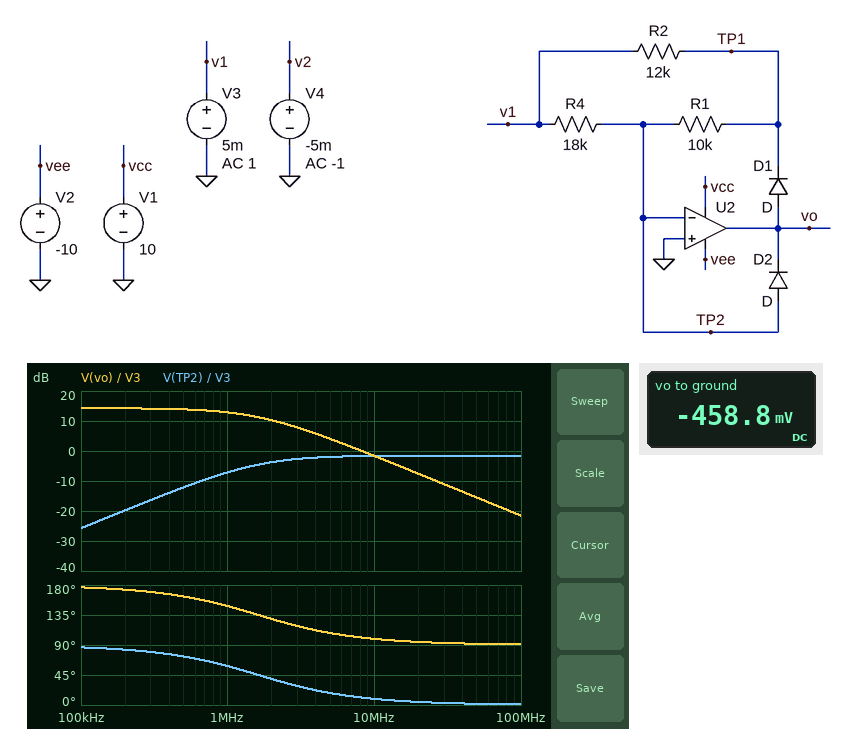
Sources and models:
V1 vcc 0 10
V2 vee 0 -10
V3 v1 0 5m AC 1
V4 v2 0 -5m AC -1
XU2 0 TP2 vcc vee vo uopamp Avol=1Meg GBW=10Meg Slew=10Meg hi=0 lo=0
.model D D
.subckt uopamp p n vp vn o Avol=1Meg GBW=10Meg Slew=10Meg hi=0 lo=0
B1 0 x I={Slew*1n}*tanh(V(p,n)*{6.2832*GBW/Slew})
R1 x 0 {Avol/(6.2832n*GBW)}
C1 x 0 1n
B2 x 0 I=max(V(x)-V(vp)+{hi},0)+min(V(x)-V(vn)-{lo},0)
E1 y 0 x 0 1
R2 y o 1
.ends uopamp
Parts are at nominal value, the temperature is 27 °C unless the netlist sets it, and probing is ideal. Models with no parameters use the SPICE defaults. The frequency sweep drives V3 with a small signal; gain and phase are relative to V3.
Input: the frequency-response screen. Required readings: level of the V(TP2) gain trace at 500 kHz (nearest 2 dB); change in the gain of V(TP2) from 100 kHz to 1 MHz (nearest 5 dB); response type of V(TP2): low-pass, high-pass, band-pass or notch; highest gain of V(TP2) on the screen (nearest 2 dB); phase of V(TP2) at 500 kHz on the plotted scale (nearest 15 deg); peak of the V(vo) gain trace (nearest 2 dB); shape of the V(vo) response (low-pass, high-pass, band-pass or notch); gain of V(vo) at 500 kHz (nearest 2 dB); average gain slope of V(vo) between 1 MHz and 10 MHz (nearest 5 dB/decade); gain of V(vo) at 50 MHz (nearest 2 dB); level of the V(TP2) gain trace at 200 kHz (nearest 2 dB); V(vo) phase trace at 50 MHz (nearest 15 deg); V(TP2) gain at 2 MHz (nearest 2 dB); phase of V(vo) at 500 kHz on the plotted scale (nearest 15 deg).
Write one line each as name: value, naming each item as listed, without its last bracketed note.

level of the V(TP2) gain trace at 500 kHz: -12 dB
change in the gain of V(TP2) from 100 kHz to 1 MHz: 20 dB
response type of V(TP2): low-pass, high-pass, band-pass or notch: high-pass
highest gain of V(TP2) on the screen: -2 dB
phase of V(TP2) at 500 kHz on the plotted scale: 75 deg
peak of the V(vo) gain trace: 14 dB
shape of the V(vo) response: low-pass
gain of V(vo) at 500 kHz: 14 dB
average gain slope of V(vo) between 1 MHz and 10 MHz: -15 dB/decade
gain of V(vo) at 50 MHz: -16 dB
level of the V(TP2) gain trace at 200 kHz: -20 dB
V(vo) phase trace at 50 MHz: 90 deg
V(TP2) gain at 2 MHz: -4 dB
phase of V(vo) at 500 kHz on the plotted scale: 165 deg
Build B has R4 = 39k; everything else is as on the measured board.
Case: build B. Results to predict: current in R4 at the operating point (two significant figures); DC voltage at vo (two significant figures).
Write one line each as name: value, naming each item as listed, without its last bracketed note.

current in R4 at the operating point: 130 nA
DC voltage at vo: -450 mV
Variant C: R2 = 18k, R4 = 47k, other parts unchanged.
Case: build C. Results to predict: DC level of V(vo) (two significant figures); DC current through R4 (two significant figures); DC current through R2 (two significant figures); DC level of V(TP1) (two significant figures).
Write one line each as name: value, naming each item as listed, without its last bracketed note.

DC level of V(vo): -440 mV
DC current through R4: 110 nA
DC current through R2: 180 nA
DC level of V(TP1): 1.8 mV
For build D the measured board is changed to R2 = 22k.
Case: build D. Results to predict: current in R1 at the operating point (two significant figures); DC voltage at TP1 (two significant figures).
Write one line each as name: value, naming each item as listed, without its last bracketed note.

current in R1 at the operating point: 160 nA
DC voltage at TP1: 1.6 mV
